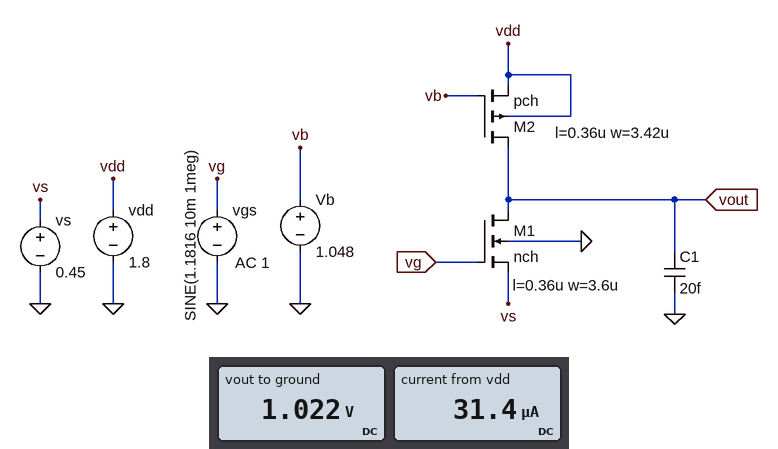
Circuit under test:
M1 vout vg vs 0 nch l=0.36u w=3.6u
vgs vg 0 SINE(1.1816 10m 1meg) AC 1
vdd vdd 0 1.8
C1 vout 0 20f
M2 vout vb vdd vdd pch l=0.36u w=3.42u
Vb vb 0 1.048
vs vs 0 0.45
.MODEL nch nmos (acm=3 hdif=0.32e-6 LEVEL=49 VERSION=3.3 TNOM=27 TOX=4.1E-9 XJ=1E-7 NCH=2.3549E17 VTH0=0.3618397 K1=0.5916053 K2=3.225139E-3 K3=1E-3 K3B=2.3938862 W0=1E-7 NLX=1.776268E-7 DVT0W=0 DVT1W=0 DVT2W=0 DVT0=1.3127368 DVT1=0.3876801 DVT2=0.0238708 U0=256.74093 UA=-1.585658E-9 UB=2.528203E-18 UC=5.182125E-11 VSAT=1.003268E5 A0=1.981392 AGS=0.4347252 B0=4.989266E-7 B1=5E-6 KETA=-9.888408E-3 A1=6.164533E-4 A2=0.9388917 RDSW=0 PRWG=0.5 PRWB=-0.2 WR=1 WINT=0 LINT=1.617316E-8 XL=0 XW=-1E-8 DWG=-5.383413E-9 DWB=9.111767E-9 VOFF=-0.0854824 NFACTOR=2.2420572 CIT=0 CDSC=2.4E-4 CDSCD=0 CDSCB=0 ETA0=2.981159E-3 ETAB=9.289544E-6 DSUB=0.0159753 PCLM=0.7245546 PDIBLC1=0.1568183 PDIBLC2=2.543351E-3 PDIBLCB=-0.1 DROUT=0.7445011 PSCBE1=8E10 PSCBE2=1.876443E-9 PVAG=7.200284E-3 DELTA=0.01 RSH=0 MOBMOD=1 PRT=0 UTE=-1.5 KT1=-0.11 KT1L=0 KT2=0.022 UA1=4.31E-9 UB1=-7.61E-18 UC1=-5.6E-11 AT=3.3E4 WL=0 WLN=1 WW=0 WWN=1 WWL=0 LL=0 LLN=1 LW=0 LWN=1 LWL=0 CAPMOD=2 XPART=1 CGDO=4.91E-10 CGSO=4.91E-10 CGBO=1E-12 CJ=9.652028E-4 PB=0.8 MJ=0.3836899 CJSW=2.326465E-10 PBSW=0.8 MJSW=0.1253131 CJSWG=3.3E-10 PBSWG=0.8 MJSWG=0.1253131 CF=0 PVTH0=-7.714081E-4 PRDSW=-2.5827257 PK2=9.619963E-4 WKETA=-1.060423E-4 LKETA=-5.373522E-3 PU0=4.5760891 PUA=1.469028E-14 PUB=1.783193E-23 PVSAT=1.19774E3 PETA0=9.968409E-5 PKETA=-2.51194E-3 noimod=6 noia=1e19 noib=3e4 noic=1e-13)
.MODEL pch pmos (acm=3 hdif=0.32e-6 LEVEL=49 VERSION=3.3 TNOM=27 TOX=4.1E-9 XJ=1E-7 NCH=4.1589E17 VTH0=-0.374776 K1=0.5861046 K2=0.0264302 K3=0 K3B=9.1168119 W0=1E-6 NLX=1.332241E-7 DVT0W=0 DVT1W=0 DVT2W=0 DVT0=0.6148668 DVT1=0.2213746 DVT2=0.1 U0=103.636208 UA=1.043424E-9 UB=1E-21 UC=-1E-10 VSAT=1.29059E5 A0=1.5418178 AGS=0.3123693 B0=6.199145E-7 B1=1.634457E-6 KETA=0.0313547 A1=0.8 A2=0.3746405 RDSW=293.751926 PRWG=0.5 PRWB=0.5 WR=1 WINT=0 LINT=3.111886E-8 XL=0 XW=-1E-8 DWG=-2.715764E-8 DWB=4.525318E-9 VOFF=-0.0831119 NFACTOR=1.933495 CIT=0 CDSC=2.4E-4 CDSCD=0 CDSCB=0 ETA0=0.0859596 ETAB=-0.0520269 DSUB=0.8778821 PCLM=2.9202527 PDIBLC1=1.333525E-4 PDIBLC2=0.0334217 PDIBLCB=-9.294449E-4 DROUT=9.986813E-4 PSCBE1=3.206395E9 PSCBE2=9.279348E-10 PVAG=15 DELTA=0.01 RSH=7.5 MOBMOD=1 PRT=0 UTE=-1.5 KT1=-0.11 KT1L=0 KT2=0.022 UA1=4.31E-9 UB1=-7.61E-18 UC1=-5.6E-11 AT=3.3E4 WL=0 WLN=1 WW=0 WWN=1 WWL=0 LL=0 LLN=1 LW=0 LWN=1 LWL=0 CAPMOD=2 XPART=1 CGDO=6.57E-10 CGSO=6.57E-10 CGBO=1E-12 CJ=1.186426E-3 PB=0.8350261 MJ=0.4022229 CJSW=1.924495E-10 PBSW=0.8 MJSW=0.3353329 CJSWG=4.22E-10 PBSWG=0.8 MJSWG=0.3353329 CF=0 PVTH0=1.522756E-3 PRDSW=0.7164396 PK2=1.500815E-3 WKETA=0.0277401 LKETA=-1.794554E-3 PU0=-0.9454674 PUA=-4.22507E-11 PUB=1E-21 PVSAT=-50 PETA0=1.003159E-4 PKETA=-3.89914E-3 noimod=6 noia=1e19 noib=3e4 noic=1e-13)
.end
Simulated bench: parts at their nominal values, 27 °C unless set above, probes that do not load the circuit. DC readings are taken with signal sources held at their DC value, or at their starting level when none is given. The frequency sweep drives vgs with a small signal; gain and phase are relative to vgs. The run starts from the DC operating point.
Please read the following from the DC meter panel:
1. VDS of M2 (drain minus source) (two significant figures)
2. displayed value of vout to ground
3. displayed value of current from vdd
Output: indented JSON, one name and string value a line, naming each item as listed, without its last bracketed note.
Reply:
{
  "VDS of M2 (drain minus source)": "-780 mV",
  "displayed value of vout to ground": "1.022 V",
  "displayed value of current from vdd": "31.4 µA"
}
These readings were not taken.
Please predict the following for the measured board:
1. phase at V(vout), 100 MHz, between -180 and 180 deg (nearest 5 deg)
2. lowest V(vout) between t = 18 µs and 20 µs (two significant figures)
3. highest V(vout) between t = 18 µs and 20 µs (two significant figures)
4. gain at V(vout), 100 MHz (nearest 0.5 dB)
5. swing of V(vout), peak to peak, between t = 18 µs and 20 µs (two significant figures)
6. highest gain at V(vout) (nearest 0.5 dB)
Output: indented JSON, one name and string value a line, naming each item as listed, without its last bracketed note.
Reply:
{
  "phase at V(vout), 100 MHz, between -180 and 180 deg": "115 deg",
  "lowest V(vout) between t = 18 µs and 20 µs": "670 mV",
  "highest V(vout) between t = 18 µs and 20 µs": "1.4 V",
  "gain at V(vout), 100 MHz": "25.0 dB",
  "swing of V(vout), peak to peak, between t = 18 µs and 20 µs": "740 mV",
  "highest gain at V(vout)": "32.5 dB"
}
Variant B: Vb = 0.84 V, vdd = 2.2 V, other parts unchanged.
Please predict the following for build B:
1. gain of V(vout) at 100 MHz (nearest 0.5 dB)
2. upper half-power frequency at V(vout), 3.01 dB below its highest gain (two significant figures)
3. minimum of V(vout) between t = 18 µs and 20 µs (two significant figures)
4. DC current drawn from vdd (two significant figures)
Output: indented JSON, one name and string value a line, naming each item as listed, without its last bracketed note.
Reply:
{
  "gain of V(vout) at 100 MHz": "-1.5 dB",
  "upper half-power frequency at V(vout), 3.01 dB below its highest gain": "1.9 GHz",
  "minimum of V(vout) between t = 18 µs and 20 µs": "2.1 V",
  "DC current drawn from vdd": "37 µA"
}
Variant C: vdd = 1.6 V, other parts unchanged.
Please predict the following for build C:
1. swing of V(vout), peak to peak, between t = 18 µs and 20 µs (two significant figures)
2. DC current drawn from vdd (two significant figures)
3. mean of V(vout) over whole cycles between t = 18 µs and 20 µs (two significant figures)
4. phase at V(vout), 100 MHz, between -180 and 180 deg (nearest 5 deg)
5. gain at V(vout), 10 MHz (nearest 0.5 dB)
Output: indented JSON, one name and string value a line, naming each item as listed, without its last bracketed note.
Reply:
{
  "swing of V(vout), peak to peak, between t = 18 µs and 20 µs": "2.2 mV",
  "DC current drawn from vdd": "4.7 µA",
  "mean of V(vout) over whole cycles between t = 18 µs and 20 µs": "460 mV",
  "phase at V(vout), 100 MHz, between -180 and 180 deg": "170 deg",
  "gain at V(vout), 10 MHz": "-19.0 dB"
}
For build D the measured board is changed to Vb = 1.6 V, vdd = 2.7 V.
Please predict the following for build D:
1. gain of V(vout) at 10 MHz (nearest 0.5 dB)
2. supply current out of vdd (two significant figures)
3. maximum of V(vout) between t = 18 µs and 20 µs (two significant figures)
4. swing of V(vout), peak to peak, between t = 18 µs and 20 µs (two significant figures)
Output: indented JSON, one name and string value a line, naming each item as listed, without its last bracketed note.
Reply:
{
  "gain of V(vout) at 10 MHz": "2.0 dB",
  "supply current out of vdd": "39 µA",
  "maximum of V(vout) between t = 18 µs and 20 µs": "2.6 V",
  "swing of V(vout), peak to peak, between t = 18 µs and 20 µs": "25 mV"
}
